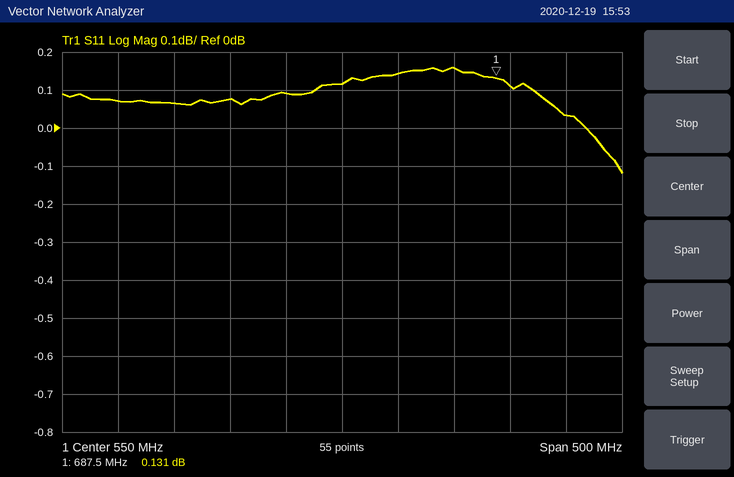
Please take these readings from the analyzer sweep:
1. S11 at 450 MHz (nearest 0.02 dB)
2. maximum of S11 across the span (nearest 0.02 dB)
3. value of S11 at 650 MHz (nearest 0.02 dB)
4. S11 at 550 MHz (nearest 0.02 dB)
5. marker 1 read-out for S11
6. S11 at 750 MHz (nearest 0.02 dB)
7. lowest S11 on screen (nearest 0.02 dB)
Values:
0.08 dB
0.16 dB
0.16 dB
0.12 dB
0.131 dB
0.04 dB
-0.12 dB
